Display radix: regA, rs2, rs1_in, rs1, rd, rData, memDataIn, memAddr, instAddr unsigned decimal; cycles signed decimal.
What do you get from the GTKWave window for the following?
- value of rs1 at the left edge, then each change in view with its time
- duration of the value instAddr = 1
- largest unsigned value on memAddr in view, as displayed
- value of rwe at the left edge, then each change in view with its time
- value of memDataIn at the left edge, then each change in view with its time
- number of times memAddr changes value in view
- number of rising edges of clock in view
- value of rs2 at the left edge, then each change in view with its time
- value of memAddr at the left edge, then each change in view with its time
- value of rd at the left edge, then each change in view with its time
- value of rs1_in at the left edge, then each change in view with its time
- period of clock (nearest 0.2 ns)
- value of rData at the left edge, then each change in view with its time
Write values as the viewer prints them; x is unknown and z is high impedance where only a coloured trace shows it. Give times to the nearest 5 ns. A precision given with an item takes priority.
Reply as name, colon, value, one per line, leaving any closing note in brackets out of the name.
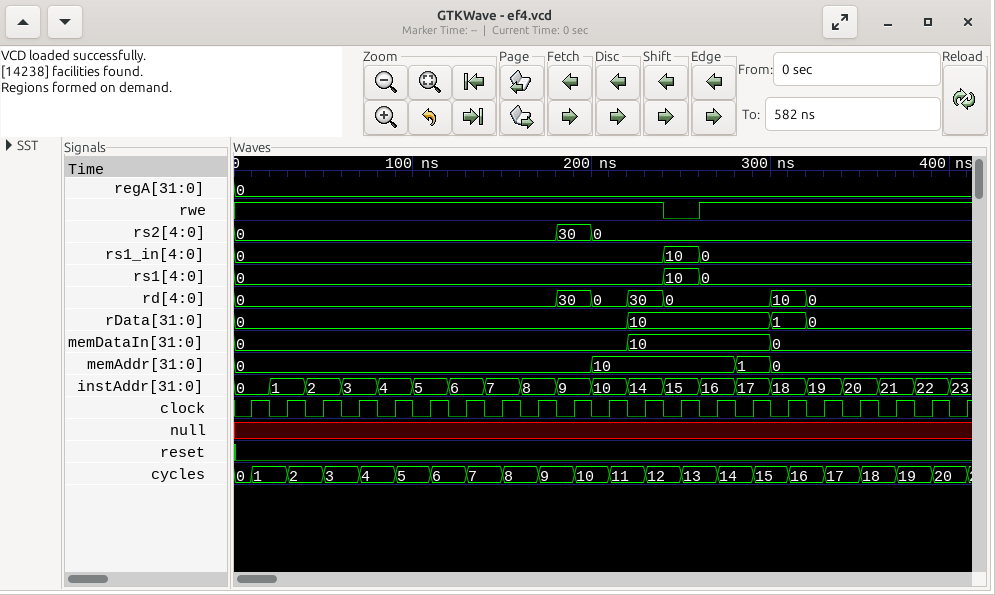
value of rs1 at the left edge, then each change in view with its time: 0, 10 at 240 ns, 0 at 260 ns
duration of the value instAddr = 1: 20 ns
largest unsigned value on memAddr in view, as displayed: 10
value of rwe at the left edge, then each change in view with its time: 1, 0 at 240 ns, 1 at 260 ns
value of memDataIn at the left edge, then each change in view with its time: 0, 10 at 220 ns, 0 at 300 ns
number of times memAddr changes value in view: 3
number of rising edges of clock in view: 21
value of rs2 at the left edge, then each change in view with its time: 0, 30 at 180 ns, 0 at 200 ns
value of memAddr at the left edge, then each change in view with its time: 0, 10 at 200 ns, 1 at 280 ns, 0 at 300 ns
value of rd at the left edge, then each change in view with its time: 0, 30 at 180 ns, 0 at 200 ns, 30 at 220 ns, 0 at 240 ns, 10 at 300 ns, 0 at 320 ns
value of rs1_in at the left edge, then each change in view with its time: 0, 10 at 240 ns, 0 at 260 ns
period of clock: 20 ns
value of rData at the left edge, then each change in view with its time: 0, 10 at 220 ns, 1 at 300 ns, 0 at 320 ns
